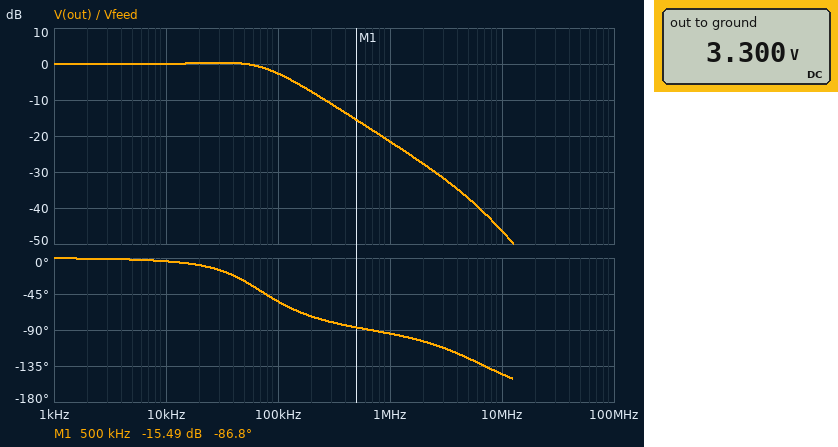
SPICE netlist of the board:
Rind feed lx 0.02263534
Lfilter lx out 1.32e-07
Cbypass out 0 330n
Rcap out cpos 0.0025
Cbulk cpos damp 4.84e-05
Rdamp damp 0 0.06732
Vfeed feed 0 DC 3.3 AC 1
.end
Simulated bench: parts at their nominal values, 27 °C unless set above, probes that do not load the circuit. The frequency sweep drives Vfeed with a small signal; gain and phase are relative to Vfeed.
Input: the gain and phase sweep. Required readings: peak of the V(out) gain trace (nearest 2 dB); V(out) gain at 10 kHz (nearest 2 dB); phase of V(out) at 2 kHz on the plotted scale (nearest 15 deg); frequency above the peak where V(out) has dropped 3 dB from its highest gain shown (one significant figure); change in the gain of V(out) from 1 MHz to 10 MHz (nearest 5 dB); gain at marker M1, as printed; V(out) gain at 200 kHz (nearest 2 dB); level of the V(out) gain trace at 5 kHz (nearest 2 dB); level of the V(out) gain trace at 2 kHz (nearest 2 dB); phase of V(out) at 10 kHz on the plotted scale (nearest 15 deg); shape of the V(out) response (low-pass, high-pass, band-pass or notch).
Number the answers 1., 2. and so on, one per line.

1. 0 dB
2. 0 dB
3. 0 deg
4. 100 kHz
5. -25 dB
6. -15.49 dB
7. -8 dB
8. 0 dB
9. 0 dB
10. 0 deg
11. low-pass
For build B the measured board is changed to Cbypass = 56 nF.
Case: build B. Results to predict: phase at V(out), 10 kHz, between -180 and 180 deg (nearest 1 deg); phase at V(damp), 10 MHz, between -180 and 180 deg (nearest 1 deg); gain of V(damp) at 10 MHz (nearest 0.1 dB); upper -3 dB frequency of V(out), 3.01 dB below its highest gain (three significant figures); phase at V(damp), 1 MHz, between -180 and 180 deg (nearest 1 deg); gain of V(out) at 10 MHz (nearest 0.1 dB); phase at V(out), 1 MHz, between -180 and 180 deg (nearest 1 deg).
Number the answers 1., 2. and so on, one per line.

1. -4 deg
2. -103 deg
3. -42.1 dB
4. 100 kHz
5. -85 deg
6. -41.7 dB
7. -88 deg
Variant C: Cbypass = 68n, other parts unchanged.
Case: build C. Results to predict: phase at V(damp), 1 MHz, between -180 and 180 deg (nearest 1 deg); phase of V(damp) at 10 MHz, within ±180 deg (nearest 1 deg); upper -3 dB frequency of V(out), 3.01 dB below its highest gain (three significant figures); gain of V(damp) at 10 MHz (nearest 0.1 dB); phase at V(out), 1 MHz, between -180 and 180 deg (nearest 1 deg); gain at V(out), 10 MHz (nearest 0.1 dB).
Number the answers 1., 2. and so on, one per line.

1. -85 deg
2. -106 deg
3. 100 kHz
4. -42.2 dB
5. -88 deg
6. -41.9 dB
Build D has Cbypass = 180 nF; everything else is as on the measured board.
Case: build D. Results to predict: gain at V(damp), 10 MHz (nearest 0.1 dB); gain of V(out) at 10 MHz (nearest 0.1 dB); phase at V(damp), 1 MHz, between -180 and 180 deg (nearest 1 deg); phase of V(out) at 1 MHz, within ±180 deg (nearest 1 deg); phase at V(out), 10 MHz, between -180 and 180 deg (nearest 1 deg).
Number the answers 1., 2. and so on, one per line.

1. -43.9 dB
2. -43.6 dB
3. -88 deg
4. -91 deg
5. -128 deg
